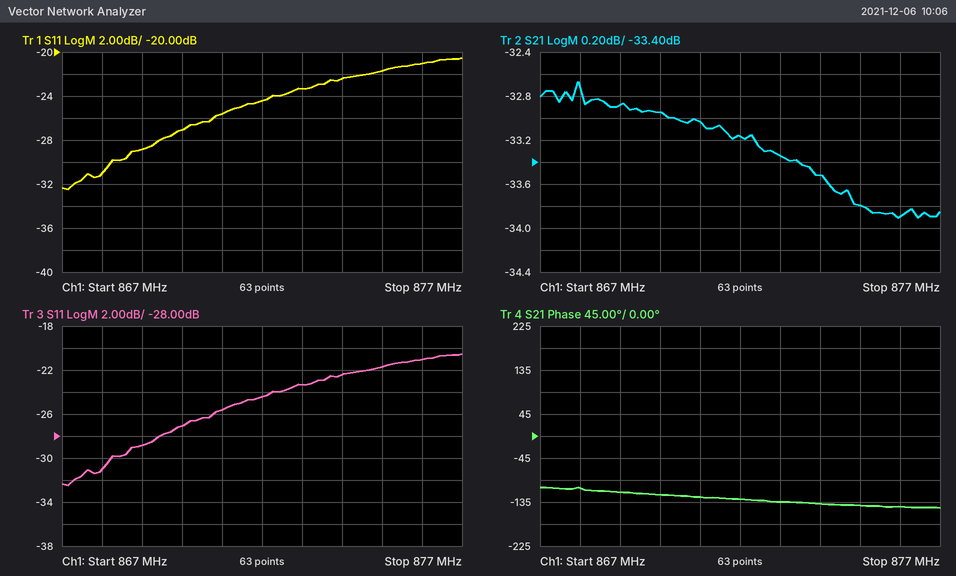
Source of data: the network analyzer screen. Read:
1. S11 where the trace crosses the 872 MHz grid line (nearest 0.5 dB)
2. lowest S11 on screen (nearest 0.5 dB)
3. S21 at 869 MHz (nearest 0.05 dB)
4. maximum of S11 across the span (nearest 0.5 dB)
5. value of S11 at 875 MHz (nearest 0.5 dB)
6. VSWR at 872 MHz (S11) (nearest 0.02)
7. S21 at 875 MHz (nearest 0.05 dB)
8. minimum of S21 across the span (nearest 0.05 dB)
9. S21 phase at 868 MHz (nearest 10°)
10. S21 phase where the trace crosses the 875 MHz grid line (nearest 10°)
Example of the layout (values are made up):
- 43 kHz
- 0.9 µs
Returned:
- -24.5 dB
- -32.5 dB
- -32.90 dB
- -20.5 dB
- -21.5 dB
- 1.12
- -33.80 dB
- -33.90 dB
- -110°
- -140°
